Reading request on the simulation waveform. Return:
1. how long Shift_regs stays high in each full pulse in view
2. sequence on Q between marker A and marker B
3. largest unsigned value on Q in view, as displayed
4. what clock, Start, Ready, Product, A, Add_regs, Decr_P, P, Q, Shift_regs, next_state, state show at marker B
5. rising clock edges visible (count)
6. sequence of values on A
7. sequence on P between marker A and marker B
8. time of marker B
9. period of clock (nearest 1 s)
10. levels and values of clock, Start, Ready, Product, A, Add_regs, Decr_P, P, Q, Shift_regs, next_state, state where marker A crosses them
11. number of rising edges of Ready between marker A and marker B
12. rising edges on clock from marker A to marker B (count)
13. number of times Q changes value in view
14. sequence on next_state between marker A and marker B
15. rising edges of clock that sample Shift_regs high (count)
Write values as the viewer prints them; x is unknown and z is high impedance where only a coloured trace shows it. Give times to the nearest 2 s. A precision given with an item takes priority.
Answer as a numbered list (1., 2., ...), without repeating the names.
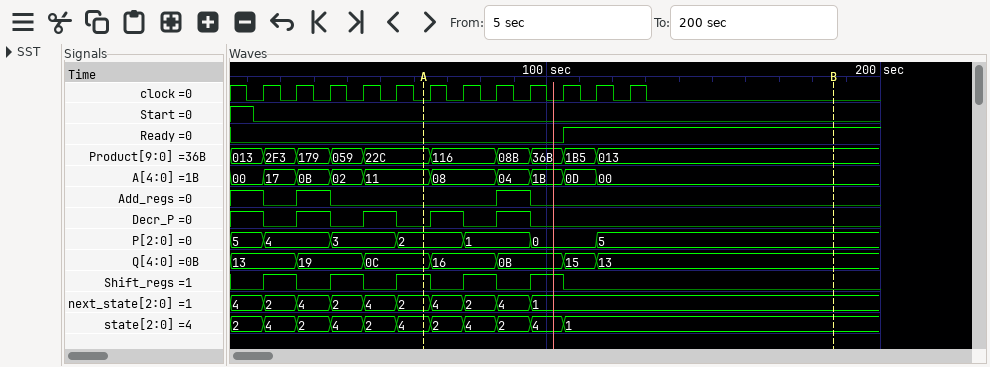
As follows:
1. 10 s, 10 s, 10 s, 10 s, 10 s
2. 0C, 16, 0B, 15, 13
3. 19
4. clock=0, Start=0, Ready=1, Product=013, A=00, Add_regs=0, Decr_P=0, P=5, Q=13, Shift_regs=0, next_state=1, state=1
5. 12
6. 00, 17, 0B, 02, 11, 08, 04, 1B, 0D, 00
7. 2, 1, 0, 5
8. 186 s
9. 10 s
10. clock=0, Start=0, Ready=0, Product=22C, A=11, Add_regs=0, Decr_P=0, P=2, Q=0C, Shift_regs=1, next_state=2, state=4
11. 1
12. 7
13. 6
14. 2, 4, 2, 4, 1
15. 5
